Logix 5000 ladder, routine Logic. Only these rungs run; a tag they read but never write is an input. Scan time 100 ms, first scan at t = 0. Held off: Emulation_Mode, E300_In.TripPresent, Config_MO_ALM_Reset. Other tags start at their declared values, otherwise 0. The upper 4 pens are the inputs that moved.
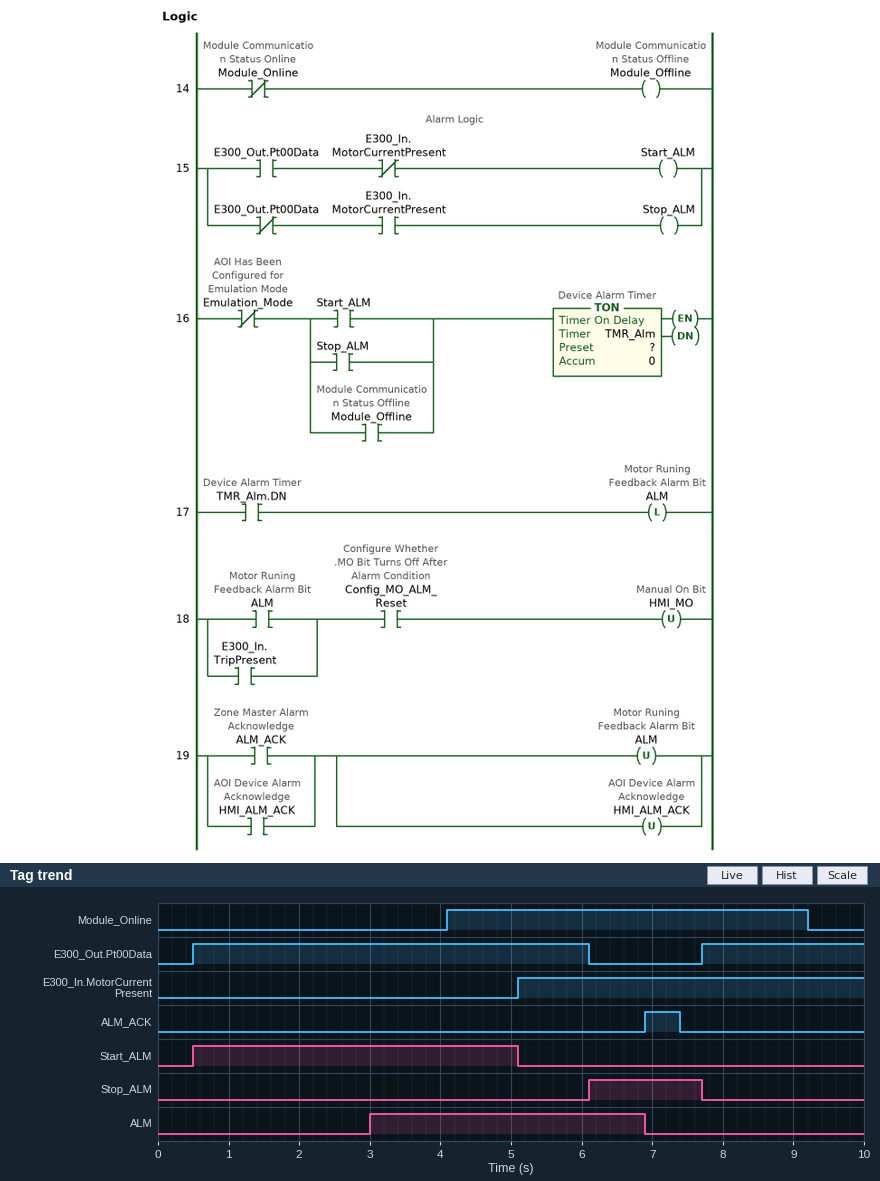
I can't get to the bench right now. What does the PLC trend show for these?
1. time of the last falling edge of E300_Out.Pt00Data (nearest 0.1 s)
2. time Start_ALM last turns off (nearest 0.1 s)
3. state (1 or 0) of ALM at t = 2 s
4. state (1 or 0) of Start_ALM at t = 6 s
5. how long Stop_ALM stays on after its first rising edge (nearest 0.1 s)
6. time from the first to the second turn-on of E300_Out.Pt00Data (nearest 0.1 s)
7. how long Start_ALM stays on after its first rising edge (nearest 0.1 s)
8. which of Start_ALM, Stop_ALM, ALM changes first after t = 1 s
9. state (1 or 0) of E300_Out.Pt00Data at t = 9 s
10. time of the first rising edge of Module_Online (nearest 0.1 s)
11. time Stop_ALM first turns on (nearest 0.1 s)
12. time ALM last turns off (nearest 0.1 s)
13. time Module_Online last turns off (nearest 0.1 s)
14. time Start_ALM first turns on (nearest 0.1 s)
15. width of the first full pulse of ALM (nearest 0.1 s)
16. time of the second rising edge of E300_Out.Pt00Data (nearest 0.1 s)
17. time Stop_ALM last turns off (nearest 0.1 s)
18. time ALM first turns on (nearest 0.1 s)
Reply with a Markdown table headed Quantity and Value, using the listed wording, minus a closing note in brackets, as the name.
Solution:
| Quantity | Value |
|---|---|
| time of the last falling edge of E300_Out.Pt00Data | 6.1 s |
| time Start_ALM last turns off | 5.1 s |
| state (1 or 0) of ALM at t = 2 s | 0 |
| state (1 or 0) of Start_ALM at t = 6 s | 0 |
| how long Stop_ALM stays on after its first rising edge | 1.6 s |
| time from the first to the second turn-on of E300_Out.Pt00Data | 7.2 s |
| how long Start_ALM stays on after its first rising edge | 4.6 s |
| which of Start_ALM, Stop_ALM, ALM changes first after t = 1 s | ALM |
| state (1 or 0) of E300_Out.Pt00Data at t = 9 s | 1 |
| time of the first rising edge of Module_Online | 4.1 s |
| time Stop_ALM first turns on | 6.1 s |
| time ALM last turns off | 6.9 s |
| time Module_Online last turns off | 9.2 s |
| time Start_ALM first turns on | 0.5 s |
| width of the first full pulse of ALM | 3.9 s |
| time of the second rising edge of E300_Out.Pt00Data | 7.7 s |
| time Stop_ALM last turns off | 7.7 s |
| time ALM first turns on | 3.0 s |
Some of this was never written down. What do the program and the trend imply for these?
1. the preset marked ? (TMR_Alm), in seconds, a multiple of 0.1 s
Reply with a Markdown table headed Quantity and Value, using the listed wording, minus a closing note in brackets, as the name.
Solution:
| Quantity | Value |
|---|---|
| the preset marked ? (TMR_Alm), in seconds, a multiple of 0.1 s | 3.0 s |
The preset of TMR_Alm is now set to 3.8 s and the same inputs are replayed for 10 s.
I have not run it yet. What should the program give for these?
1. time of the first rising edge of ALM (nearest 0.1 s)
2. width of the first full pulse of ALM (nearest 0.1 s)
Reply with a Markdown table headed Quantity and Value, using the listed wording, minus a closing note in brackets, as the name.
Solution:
| Quantity | Value |
|---|---|
| time of the first rising edge of ALM | 3.8 s |
| width of the first full pulse of ALM | 3.1 s |
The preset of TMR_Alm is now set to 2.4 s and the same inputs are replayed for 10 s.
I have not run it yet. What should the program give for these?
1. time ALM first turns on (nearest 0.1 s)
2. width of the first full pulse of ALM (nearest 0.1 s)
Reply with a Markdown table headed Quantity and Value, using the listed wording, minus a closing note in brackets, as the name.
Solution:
| Quantity | Value |
|---|---|
| time ALM first turns on | 2.4 s |
| width of the first full pulse of ALM | 4.5 s |
